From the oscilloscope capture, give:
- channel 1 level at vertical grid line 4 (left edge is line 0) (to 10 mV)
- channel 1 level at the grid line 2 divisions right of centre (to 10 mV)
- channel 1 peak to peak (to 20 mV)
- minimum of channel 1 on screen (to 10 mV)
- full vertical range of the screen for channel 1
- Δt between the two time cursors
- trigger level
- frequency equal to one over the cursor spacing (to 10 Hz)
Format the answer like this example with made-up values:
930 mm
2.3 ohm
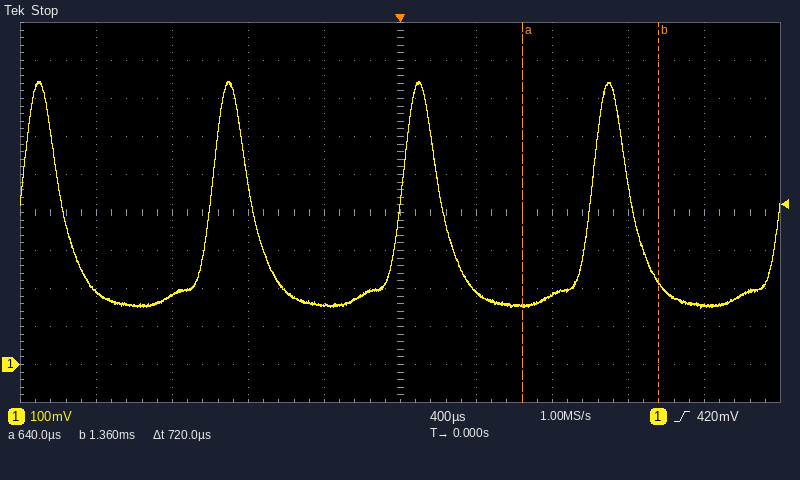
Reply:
160 mV
180 mV
600 mV
150 mV
1 V
720 µs
420 mV
1.39 kHz
